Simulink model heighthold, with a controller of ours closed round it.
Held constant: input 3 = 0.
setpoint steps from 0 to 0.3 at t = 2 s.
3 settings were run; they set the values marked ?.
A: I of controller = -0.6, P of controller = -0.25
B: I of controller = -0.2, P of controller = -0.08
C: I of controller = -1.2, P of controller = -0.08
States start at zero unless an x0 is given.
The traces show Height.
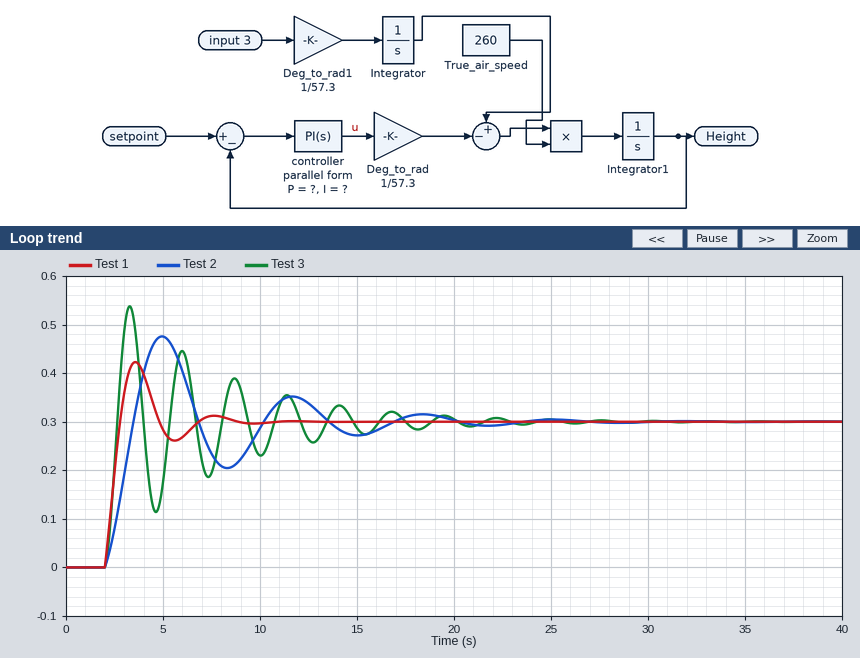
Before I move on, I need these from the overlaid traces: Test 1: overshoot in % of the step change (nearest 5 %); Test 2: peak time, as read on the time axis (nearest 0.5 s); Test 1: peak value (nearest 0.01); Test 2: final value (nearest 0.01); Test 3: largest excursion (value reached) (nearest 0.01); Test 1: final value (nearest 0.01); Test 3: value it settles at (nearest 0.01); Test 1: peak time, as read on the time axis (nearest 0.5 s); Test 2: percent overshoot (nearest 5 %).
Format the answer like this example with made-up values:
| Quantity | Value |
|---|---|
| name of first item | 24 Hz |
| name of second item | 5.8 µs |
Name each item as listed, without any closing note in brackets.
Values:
| Quantity | Value |
|---|---|
| Test 1: overshoot in % of the step change | 40 % |
| Test 2: peak time, as read on the time axis | 5.0 s |
| Test 1: peak value | 0.42 |
| Test 2: final value | 0.30 |
| Test 3: largest excursion (value reached) | 0.54 |
| Test 1: final value | 0.30 |
| Test 3: value it settles at | 0.30 |
| Test 1: peak time, as read on the time axis | 3.5 s |
| Test 2: percent overshoot | 60 % |
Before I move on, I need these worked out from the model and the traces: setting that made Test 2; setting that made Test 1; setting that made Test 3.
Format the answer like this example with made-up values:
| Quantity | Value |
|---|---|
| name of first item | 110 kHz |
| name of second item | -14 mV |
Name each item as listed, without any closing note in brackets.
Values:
| Quantity | Value |
|---|---|
| setting that made Test 2 | B |
| setting that made Test 1 | A |
| setting that made Test 3 | C |
